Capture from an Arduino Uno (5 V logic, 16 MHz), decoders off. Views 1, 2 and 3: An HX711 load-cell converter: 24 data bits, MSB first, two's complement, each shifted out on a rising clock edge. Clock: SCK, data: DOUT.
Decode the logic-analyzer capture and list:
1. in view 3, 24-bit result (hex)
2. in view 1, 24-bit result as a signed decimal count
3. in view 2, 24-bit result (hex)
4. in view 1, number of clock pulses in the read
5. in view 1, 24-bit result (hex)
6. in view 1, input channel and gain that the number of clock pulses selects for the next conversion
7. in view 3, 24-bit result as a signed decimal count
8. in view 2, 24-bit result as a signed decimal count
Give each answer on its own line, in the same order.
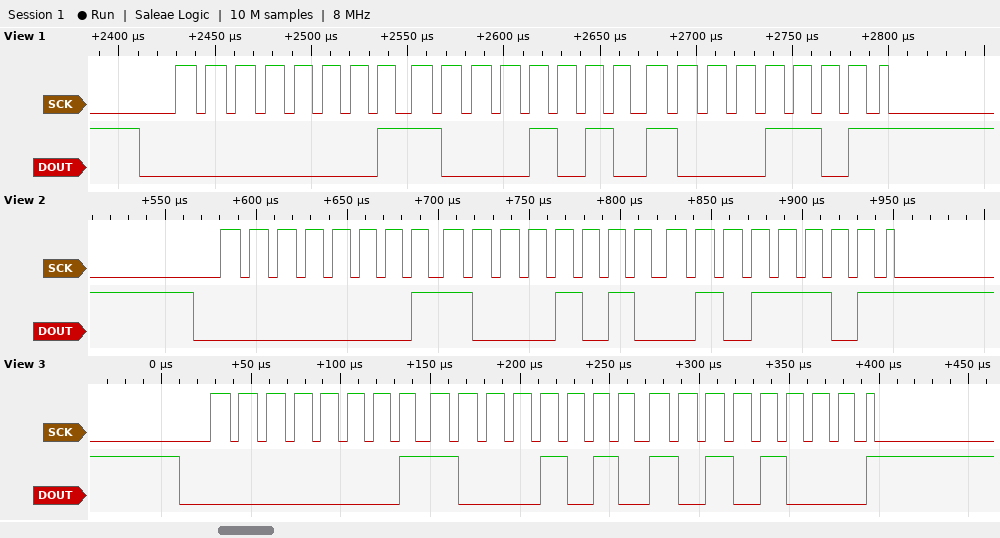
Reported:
0x018AA8
101005
0x018A5D
25
0x018A8D
channel A, gain 128
101032
100957
